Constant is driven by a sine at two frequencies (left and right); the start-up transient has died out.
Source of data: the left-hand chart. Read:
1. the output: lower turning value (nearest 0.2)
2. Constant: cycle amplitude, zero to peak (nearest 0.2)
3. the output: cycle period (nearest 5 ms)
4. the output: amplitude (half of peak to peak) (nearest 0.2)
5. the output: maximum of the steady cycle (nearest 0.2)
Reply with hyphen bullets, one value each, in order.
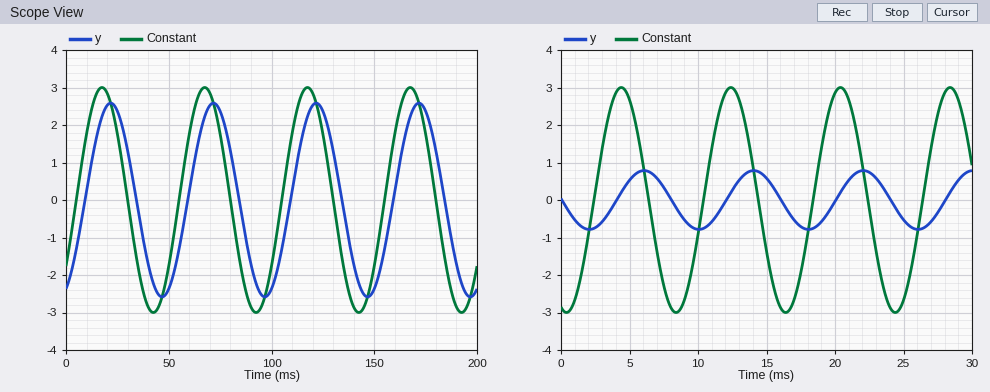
- -2.6
- 3.0
- 50 ms
- 2.6
- 2.6
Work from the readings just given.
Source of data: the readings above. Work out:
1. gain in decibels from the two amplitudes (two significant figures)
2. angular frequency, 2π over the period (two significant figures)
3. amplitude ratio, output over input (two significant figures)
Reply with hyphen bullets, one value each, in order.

- -1.2 dB
- 0.13 rad/ms
- 0.87
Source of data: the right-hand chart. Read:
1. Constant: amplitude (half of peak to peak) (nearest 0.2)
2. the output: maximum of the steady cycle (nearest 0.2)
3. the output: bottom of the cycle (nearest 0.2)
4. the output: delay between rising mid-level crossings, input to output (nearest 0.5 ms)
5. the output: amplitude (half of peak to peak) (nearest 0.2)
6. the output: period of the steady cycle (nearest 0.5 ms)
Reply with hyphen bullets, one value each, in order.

- 3.0
- 0.8
- -0.8
- 1.5 ms
- 0.8
- 8.0 ms
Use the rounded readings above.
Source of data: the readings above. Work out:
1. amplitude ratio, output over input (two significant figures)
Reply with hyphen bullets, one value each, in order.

- 0.27
